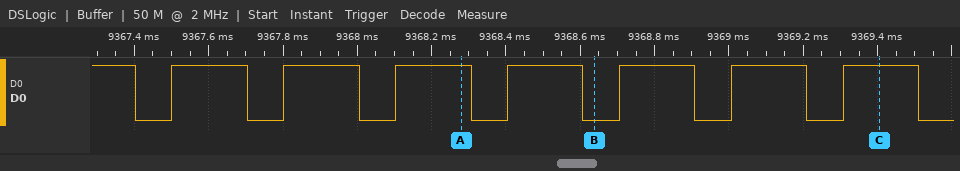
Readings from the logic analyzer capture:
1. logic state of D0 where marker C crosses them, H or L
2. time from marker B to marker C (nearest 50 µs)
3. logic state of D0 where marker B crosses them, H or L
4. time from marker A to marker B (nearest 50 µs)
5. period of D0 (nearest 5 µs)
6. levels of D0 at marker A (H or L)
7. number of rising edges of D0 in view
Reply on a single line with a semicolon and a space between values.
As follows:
D0=H; 750 µs; D0=L; 350 µs; 300 µs; D0=H; 7
